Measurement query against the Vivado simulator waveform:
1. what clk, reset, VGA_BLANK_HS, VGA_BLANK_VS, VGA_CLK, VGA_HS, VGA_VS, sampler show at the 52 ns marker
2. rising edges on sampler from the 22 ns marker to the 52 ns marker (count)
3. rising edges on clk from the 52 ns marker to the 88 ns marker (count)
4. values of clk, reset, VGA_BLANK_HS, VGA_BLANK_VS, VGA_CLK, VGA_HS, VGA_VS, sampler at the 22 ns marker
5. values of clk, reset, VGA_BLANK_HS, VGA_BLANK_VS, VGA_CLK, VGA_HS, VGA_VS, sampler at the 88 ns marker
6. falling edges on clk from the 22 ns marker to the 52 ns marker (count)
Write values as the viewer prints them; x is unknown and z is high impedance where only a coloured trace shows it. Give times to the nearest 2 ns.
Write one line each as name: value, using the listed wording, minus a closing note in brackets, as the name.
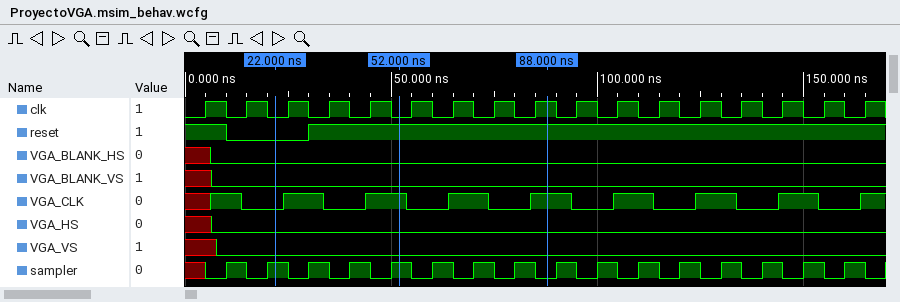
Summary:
what clk, reset, VGA_BLANK_HS, VGA_BLANK_VS, VGA_CLK, VGA_HS, VGA_VS, sampler show at the 52 ns marker: clk=0, reset=1, VGA_BLANK_HS=0, VGA_BLANK_VS=0, VGA_CLK=1, VGA_HS=0, VGA_VS=0, sampler=1
rising edges on sampler from the 22 ns marker to the 52 ns marker: 3
rising edges on clk from the 52 ns marker to the 88 ns marker: 4
values of clk, reset, VGA_BLANK_HS, VGA_BLANK_VS, VGA_CLK, VGA_HS, VGA_VS, sampler at the 22 ns marker: clk=0, reset=0, VGA_BLANK_HS=0, VGA_BLANK_VS=0, VGA_CLK=0, VGA_HS=0, VGA_VS=0, sampler=1
values of clk, reset, VGA_BLANK_HS, VGA_BLANK_VS, VGA_CLK, VGA_HS, VGA_VS, sampler at the 88 ns marker: clk=1, reset=1, VGA_BLANK_HS=0, VGA_BLANK_VS=0, VGA_CLK=1, VGA_HS=0, VGA_VS=0, sampler=0
falling edges on clk from the 22 ns marker to the 52 ns marker: 3
